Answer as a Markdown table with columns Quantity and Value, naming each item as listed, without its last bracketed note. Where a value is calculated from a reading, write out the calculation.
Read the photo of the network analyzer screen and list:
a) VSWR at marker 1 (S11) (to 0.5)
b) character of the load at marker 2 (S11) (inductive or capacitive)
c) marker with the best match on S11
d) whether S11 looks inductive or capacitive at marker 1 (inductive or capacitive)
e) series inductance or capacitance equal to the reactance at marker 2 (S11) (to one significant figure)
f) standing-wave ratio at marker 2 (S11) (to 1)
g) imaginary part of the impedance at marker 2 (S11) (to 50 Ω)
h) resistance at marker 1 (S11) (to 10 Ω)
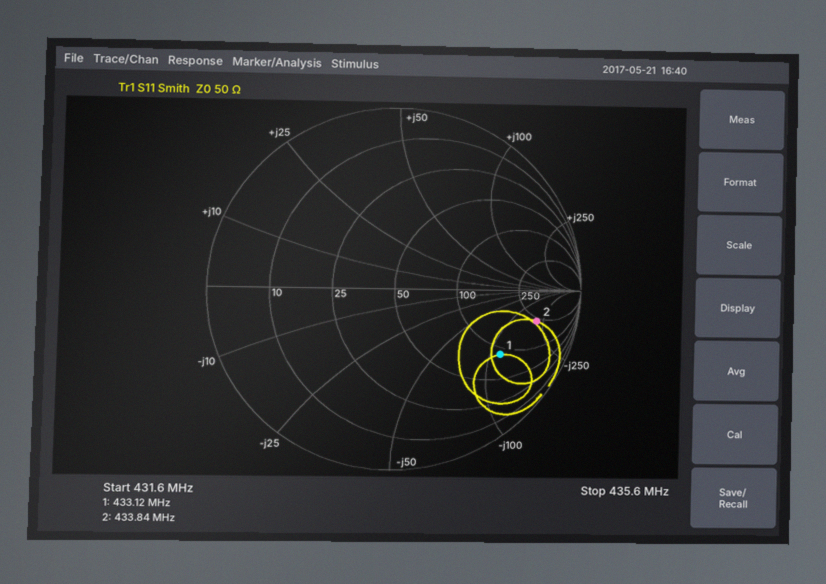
| Quantity | Value |
|---|---|
| VSWR at marker 1 (S11) | 5.0 |
| character of the load at marker 2 (S11) | capacitive |
| marker with the best match on S11 | marker 1 |
| whether S11 looks inductive or capacitive at marker 1 | capacitive |
| series inductance or capacitance equal to the reactance at marker 2 (S11) | C = 1/(2π × 433.84 MHz × 200 Ω) ≈ 2 pF |
| standing-wave ratio at marker 2 (S11) | 8 |
| imaginary part of the impedance at marker 2 (S11) | -200 Ω |
| resistance at marker 1 (S11) | 90 Ω |
